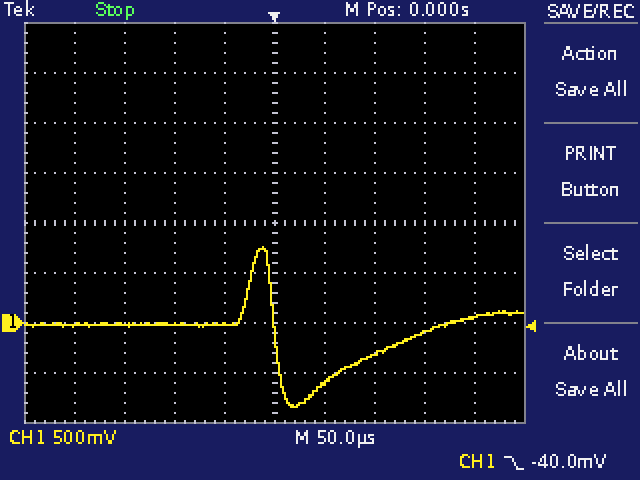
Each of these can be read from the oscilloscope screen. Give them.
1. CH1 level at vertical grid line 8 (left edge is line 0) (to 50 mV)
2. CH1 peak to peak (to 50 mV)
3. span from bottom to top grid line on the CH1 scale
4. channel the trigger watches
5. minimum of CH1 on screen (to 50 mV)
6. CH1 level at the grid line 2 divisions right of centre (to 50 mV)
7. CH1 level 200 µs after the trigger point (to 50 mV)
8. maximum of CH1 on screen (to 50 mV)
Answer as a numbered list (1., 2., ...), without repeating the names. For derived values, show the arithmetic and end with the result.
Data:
1. -100 mV
2. 750 mV − (-850 mV) = 1.60 V
3. 4 V
4. CH1
5. -850 mV
6. -300 mV
7. 50 mV
8. 750 mV
